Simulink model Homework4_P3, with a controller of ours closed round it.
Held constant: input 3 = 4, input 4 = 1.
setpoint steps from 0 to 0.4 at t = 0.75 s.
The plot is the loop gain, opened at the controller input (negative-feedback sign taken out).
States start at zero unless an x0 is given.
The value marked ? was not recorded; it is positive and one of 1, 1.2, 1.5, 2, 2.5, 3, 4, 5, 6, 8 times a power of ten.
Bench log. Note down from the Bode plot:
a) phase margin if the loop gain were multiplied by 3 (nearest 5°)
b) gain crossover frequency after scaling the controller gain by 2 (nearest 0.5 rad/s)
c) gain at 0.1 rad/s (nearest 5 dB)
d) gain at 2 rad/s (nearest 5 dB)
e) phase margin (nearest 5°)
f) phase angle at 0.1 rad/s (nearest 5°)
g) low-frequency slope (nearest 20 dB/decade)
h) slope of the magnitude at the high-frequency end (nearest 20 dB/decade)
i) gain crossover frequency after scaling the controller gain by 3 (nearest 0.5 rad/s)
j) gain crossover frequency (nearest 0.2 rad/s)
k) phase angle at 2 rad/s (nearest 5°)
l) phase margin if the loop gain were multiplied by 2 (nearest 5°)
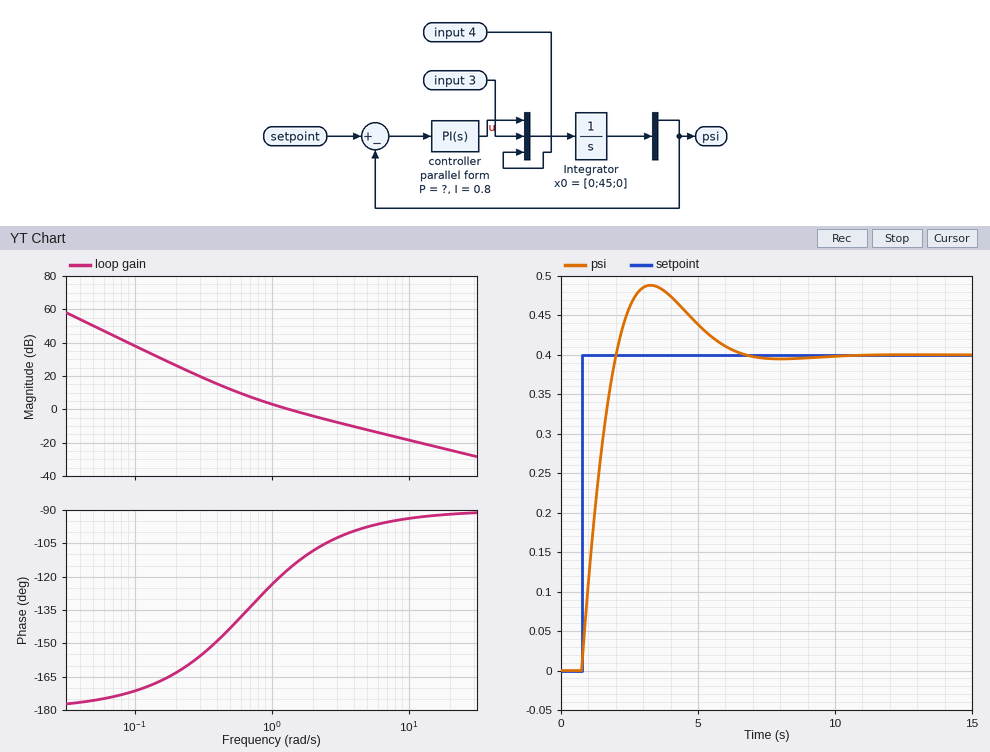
80°
2.5 rad/s
40 dB
-5 dB
65°
-170°
-40 dB/decade
-20 dB/decade
3.5 rad/s
1.4 rad/s
-110°
75°
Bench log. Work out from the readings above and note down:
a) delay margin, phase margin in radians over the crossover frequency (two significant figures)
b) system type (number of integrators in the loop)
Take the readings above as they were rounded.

0.81 s
2
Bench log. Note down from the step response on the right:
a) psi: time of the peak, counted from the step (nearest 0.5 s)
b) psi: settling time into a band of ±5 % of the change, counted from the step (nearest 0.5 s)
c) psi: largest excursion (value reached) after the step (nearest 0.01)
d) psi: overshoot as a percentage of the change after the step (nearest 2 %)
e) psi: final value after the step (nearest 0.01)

2.5 s
5.0 s
0.49
22 %
0.40
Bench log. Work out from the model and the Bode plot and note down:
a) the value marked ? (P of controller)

1.2
